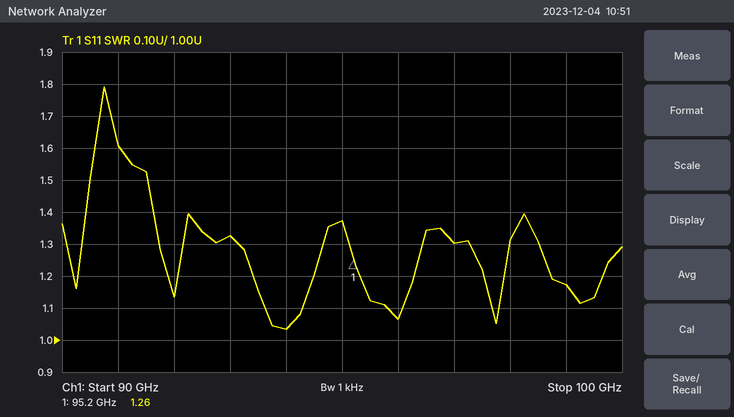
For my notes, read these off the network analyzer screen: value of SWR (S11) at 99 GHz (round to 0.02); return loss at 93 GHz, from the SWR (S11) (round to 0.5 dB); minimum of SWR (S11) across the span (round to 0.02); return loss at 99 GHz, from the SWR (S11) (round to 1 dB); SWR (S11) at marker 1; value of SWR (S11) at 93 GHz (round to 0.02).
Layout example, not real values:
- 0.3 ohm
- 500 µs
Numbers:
- 1.18
- 17.0 dB
- 1.04
- 22 dB
- 1.26
- 1.32
